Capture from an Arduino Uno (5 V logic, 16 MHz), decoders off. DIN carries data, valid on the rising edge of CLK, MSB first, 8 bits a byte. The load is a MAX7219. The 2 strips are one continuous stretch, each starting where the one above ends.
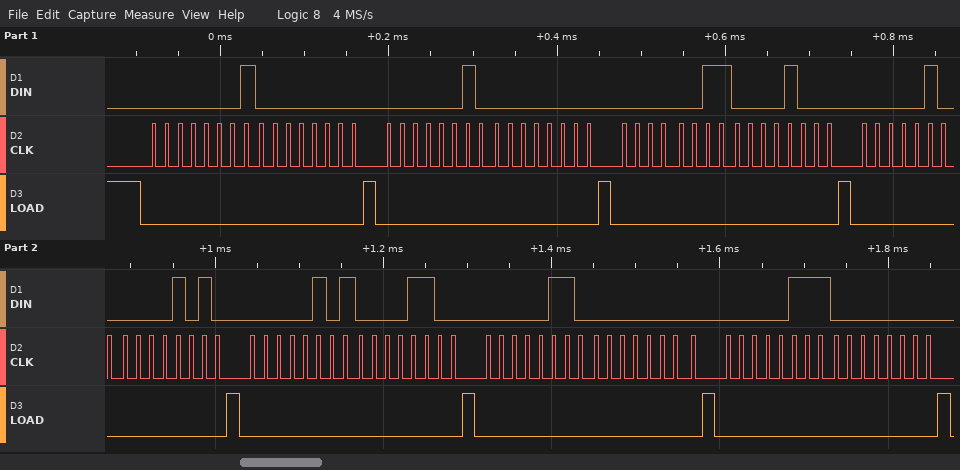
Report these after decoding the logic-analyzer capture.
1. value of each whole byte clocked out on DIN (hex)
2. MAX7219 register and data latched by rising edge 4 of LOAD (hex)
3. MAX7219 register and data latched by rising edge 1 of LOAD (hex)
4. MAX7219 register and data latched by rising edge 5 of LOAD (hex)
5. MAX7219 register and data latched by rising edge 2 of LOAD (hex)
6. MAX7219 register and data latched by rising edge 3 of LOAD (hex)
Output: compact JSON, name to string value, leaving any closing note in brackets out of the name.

{"value of each whole byte clocked out on DIN": "01 00 02 00 03 08 04 0A 05 0C 06 00 07 00", "MAX7219 register and data latched by rising edge 4 of LOAD": "register 0x4, data 0x0A", "MAX7219 register and data latched by rising edge 1 of LOAD": "register 0x1, data 0x00", "MAX7219 register and data latched by rising edge 5 of LOAD": "register 0x5, data 0x0C", "MAX7219 register and data latched by rising edge 2 of LOAD": "register 0x2, data 0x00", "MAX7219 register and data latched by rising edge 3 of LOAD": "register 0x3, data 0x08"}
